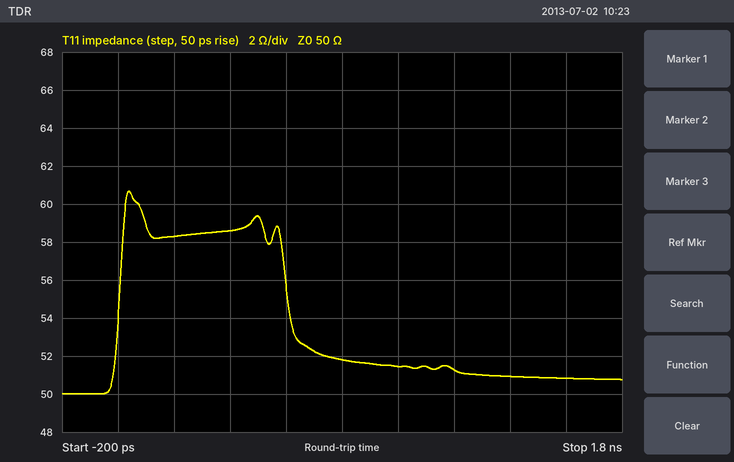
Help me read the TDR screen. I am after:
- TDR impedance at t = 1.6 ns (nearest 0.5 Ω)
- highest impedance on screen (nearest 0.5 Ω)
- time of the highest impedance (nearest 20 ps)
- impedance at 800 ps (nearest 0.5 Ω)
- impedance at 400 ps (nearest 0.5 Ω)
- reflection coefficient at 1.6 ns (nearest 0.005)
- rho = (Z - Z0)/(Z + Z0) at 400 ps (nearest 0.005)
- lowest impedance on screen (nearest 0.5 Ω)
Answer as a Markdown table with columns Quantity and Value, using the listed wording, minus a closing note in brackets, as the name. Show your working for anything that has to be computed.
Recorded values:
| Quantity | Value |
|---|---|
| TDR impedance at t = 1.6 ns | 51.0 Ω |
| highest impedance on screen | 60.5 Ω |
| time of the highest impedance | 40 ps |
| impedance at 800 ps | 52.0 Ω |
| impedance at 400 ps | 58.5 Ω |
| reflection coefficient at 1.6 ns | (51 − 50)/(51 + 50) ≈ +0.010 |
| rho = (Z - Z0)/(Z + Z0) at 400 ps | (58.5 − 50)/(58.5 + 50) ≈ +0.0783, so +0.080 to the nearest 0.005 |
| lowest impedance on screen | 50.0 Ω |
